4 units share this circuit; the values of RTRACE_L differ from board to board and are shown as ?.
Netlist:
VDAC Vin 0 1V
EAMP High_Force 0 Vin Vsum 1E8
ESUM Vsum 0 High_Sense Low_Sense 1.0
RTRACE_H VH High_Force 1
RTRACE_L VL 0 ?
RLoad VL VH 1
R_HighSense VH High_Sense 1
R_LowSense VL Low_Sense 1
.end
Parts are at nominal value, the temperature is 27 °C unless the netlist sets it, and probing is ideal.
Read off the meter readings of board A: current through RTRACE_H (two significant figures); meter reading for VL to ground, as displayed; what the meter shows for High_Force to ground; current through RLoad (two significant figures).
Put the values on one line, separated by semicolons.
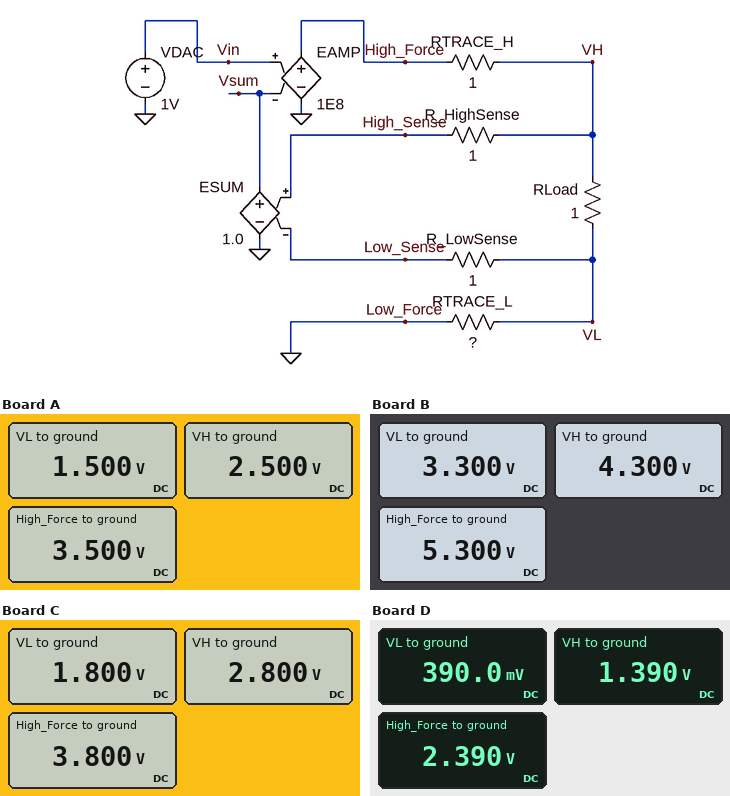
1.0 A; 1.500 V; 3.500 V; 1.0 A
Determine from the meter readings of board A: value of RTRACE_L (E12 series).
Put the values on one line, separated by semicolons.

1.5 Ω
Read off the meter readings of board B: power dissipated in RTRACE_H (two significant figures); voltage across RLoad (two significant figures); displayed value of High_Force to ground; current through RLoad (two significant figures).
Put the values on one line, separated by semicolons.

1.0 W; 1.0 V; 5.300 V; 1.0 A
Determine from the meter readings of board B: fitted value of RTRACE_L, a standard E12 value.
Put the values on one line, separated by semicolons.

3.3 Ω
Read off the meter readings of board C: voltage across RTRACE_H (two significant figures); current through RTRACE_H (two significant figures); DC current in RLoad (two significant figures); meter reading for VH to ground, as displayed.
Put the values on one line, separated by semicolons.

1.0 V; 1.0 A; 1.0 A; 2.800 V
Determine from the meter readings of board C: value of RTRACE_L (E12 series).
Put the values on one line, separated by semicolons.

1.8 Ω
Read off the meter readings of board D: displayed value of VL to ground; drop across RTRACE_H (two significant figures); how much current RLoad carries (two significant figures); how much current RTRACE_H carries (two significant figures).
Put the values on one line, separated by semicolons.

390.0 mV; 1.0 V; 1.0 A; 1.0 A
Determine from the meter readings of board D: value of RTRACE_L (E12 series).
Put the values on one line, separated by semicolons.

0.39 Ω
